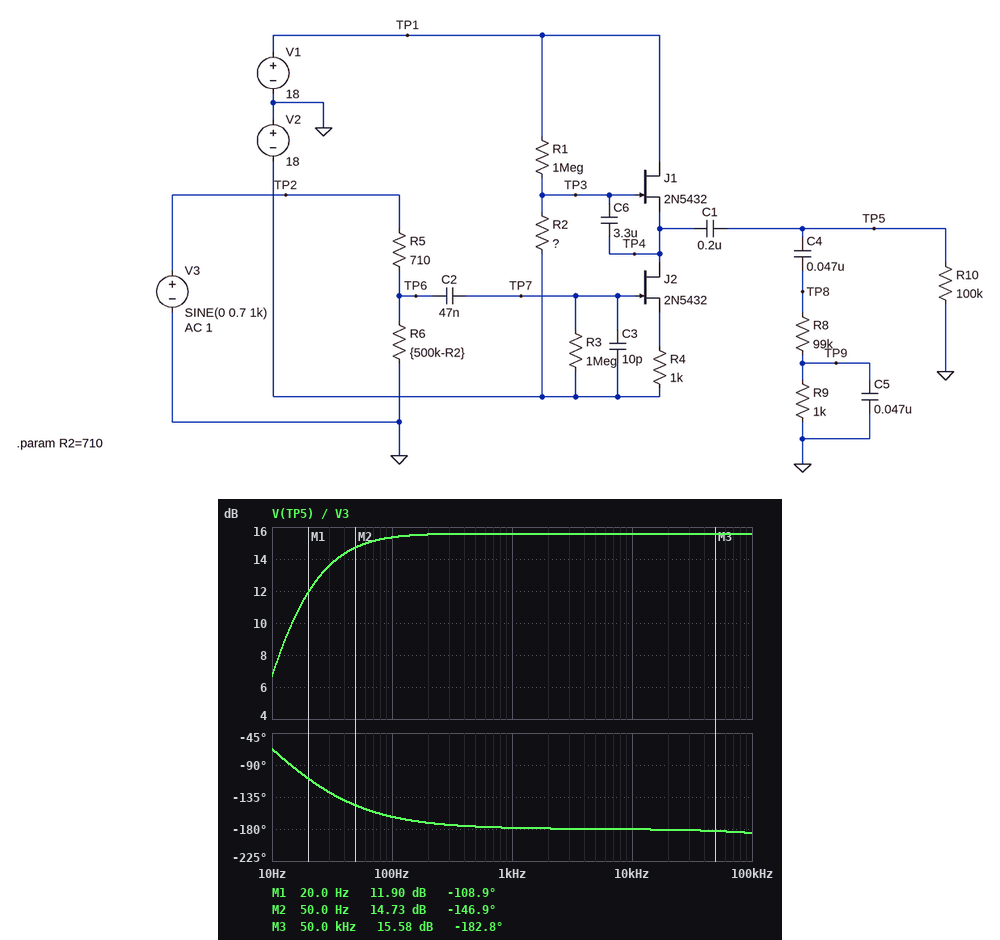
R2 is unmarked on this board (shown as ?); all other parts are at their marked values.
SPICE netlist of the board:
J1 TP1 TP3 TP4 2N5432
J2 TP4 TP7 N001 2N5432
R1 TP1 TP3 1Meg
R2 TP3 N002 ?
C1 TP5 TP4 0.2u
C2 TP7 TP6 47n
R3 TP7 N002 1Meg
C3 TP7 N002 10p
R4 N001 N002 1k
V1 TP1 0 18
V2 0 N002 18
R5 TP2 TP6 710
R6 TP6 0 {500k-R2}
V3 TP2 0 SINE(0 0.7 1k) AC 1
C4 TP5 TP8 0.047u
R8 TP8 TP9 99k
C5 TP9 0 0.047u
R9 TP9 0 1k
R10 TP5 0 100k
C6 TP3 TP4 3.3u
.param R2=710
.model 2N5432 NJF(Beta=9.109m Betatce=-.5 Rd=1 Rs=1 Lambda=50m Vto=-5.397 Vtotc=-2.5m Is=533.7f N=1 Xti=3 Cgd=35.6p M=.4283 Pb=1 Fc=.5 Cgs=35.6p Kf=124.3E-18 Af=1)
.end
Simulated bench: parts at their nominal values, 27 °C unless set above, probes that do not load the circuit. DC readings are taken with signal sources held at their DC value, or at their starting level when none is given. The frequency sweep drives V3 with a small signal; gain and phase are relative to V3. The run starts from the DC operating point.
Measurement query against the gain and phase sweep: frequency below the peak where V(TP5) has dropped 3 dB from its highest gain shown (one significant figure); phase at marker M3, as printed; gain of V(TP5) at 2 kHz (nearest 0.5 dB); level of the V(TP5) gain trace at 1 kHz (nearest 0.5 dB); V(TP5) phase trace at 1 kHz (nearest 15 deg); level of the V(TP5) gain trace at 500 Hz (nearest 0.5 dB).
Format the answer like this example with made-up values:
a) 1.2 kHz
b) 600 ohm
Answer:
a) 20 Hz
b) -182.8 deg
c) 15.5 dB
d) 15.5 dB
e) -180 deg
f) 15.5 dB
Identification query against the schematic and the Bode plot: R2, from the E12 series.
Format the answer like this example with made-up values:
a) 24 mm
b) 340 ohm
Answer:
a) 560 kΩ
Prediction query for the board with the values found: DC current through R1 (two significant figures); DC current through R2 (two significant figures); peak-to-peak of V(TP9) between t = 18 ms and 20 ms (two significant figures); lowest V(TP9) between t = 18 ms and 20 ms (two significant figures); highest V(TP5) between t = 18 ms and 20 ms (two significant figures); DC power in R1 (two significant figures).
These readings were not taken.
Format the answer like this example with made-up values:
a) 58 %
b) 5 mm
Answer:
a) 23 µA
b) 23 µA
c) 81 mV
d) -40 mV
e) 4.2 V
f) 530 µW
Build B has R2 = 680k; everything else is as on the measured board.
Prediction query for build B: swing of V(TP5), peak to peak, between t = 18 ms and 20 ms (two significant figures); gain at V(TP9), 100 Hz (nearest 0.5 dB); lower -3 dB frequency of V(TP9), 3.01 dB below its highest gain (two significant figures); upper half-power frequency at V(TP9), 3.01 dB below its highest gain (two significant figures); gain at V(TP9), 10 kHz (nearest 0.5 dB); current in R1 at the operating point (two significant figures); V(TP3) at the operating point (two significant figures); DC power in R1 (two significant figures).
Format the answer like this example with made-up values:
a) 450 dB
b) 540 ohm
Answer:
a) 8.2 V
b) -25.5 dB
c) 43 Hz
d) 3.5 kHz
e) -34.5 dB
f) 21 µA
g) -3.4 V
h) 460 µW
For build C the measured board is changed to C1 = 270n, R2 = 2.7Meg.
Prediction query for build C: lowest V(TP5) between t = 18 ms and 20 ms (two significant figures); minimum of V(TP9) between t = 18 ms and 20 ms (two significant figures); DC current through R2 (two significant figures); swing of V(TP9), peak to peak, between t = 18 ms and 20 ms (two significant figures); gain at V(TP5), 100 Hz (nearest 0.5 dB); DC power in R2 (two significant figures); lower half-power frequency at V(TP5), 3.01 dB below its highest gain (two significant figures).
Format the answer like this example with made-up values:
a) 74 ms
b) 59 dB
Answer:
a) -3.0 V
b) -29 mV
c) 9.7 µA
d) 58 mV
e) 12.5 dB
f) 260 µW
g) 10 Hz
